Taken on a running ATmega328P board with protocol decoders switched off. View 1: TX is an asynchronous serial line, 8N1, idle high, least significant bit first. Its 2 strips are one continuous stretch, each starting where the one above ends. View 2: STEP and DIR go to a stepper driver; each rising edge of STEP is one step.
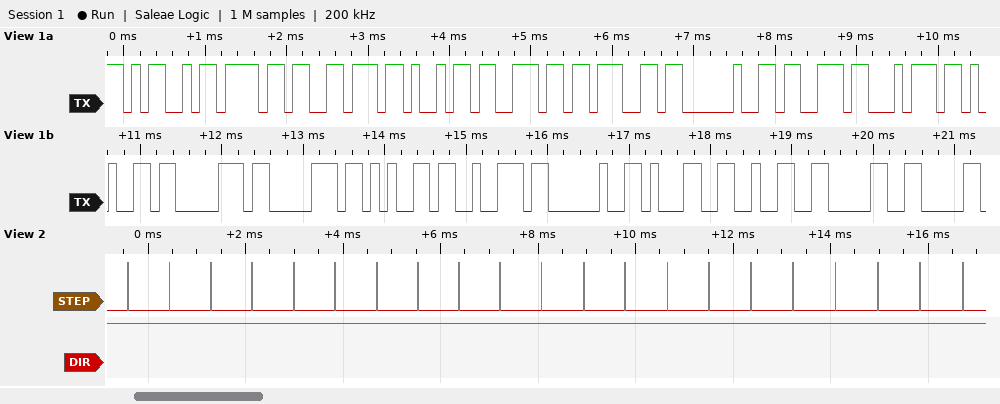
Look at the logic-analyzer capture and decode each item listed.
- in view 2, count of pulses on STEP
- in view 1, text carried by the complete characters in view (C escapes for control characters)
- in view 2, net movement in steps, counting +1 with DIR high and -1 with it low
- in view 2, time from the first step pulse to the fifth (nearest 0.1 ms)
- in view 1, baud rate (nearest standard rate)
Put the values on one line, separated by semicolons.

21; "Moving stepper 120"; +21; 3.4 ms; 9600 baud
